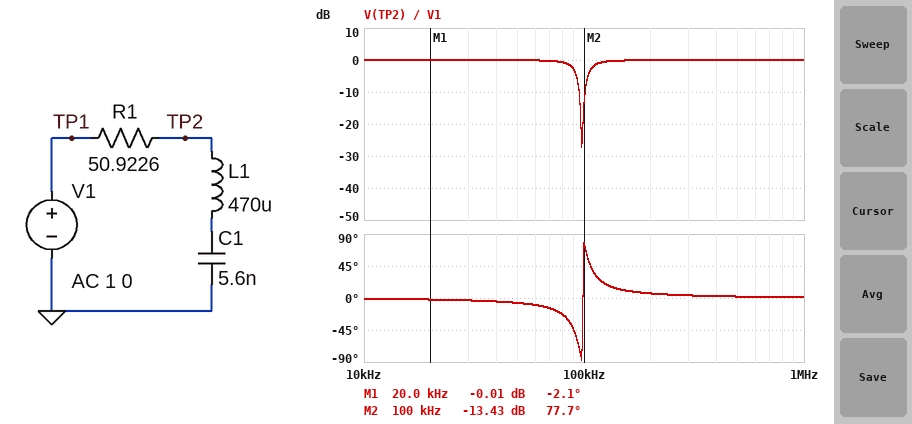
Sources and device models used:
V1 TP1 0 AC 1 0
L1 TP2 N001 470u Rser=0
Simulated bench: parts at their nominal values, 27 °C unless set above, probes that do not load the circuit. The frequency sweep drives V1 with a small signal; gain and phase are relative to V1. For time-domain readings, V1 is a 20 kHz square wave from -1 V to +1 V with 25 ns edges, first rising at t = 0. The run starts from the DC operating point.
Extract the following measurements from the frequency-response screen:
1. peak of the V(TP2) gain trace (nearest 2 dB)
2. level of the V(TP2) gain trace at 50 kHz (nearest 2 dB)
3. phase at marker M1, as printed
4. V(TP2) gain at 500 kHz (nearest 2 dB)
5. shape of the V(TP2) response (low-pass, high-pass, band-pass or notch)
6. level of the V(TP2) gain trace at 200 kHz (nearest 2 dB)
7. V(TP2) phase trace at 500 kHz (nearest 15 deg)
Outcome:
0 dB
0 dB
-2.1 deg
0 dB
notch
0 dB
0 deg
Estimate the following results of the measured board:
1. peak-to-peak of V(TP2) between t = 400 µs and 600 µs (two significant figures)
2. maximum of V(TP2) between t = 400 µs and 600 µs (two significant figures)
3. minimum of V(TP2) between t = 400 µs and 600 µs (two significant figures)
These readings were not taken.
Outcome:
2.6 V
1.3 V
-1.3 V
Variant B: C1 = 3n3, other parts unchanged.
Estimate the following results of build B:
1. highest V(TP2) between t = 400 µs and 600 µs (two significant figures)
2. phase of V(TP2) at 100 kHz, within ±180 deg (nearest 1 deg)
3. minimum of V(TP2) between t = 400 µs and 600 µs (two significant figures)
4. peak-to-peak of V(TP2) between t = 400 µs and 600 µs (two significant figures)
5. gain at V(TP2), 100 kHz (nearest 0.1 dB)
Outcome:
1.2 V
-15 deg
-1.2 V
2.3 V
-0.3 dB
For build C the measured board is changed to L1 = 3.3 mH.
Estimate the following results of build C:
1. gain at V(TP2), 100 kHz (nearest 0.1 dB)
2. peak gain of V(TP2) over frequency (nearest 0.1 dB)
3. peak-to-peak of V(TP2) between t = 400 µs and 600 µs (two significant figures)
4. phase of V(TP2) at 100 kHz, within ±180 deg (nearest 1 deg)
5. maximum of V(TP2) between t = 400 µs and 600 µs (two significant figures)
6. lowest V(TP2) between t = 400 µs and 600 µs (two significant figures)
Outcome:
0 dB
0 dB
2.1 V
2 deg
1.1 V
-1.1 V
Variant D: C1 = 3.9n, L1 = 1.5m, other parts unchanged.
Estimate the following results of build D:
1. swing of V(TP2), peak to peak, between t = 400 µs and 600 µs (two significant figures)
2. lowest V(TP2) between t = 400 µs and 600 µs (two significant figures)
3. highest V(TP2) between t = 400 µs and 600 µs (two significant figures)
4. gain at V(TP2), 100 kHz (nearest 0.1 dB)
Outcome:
2.4 V
-1.2 V
1.2 V
0 dB
